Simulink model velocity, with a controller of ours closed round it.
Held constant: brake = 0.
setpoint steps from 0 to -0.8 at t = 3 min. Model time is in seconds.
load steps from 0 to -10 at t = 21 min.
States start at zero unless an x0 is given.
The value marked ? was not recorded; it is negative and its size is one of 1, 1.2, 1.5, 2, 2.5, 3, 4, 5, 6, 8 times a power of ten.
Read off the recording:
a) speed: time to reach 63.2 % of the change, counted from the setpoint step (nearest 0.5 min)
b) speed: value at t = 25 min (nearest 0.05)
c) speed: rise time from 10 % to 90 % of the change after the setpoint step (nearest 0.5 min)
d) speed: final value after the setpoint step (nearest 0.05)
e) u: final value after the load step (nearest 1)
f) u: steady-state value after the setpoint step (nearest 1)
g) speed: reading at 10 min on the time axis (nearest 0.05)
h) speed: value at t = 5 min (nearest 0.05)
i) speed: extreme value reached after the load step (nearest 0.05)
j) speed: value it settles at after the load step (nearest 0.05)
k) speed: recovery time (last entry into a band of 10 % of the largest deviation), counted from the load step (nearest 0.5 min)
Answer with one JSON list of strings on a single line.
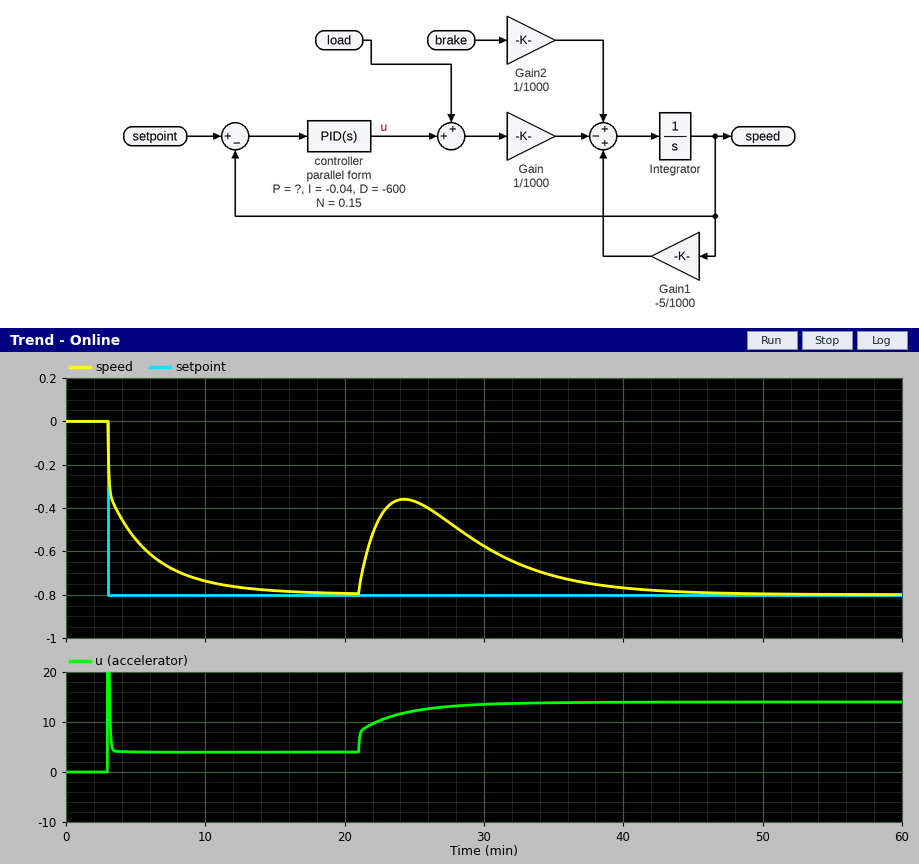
["1.5 min", "-0.35", "6.0 min", "-0.80", "14", "4", "-0.75", "-0.55", "-0.35", "-0.80", "17.5 min"]
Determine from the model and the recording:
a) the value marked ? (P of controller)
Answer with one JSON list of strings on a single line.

["-12"]
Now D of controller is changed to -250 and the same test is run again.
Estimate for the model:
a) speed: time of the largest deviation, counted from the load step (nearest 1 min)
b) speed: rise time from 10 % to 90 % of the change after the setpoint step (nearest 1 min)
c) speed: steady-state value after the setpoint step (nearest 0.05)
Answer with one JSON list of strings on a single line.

["3 min", "5 min", "-0.80"]
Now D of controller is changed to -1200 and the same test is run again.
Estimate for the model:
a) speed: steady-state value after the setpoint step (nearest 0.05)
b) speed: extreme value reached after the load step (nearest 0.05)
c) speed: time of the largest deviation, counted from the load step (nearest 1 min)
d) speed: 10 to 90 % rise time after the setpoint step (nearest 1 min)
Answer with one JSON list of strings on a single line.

["-0.80", "-0.40", "4 min", "7 min"]
